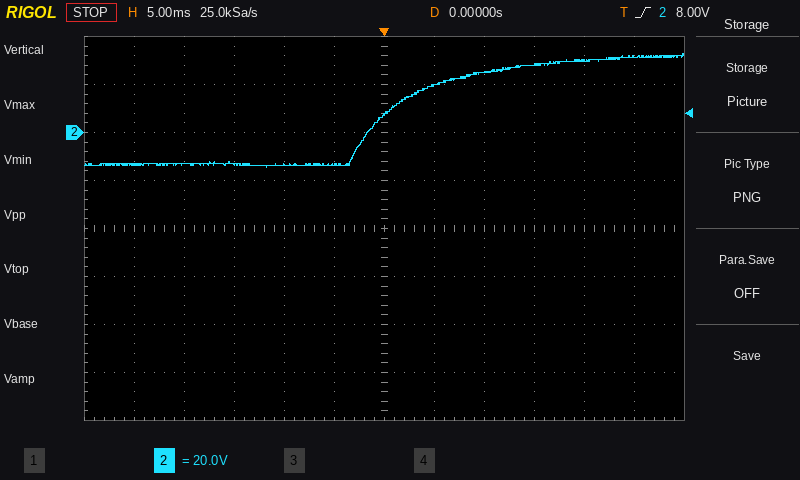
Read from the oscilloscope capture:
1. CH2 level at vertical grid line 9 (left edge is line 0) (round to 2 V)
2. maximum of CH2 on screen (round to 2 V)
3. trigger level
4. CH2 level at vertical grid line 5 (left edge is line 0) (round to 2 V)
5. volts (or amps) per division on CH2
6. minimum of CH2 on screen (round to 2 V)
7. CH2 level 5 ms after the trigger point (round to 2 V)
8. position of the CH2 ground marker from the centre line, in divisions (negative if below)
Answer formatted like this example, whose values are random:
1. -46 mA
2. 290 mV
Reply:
1. 28 V
2. 32 V
3. 8.00 V
4. -14 V
5. 20 V
6. -14 V
7. 20 V
8. +2.0 div
